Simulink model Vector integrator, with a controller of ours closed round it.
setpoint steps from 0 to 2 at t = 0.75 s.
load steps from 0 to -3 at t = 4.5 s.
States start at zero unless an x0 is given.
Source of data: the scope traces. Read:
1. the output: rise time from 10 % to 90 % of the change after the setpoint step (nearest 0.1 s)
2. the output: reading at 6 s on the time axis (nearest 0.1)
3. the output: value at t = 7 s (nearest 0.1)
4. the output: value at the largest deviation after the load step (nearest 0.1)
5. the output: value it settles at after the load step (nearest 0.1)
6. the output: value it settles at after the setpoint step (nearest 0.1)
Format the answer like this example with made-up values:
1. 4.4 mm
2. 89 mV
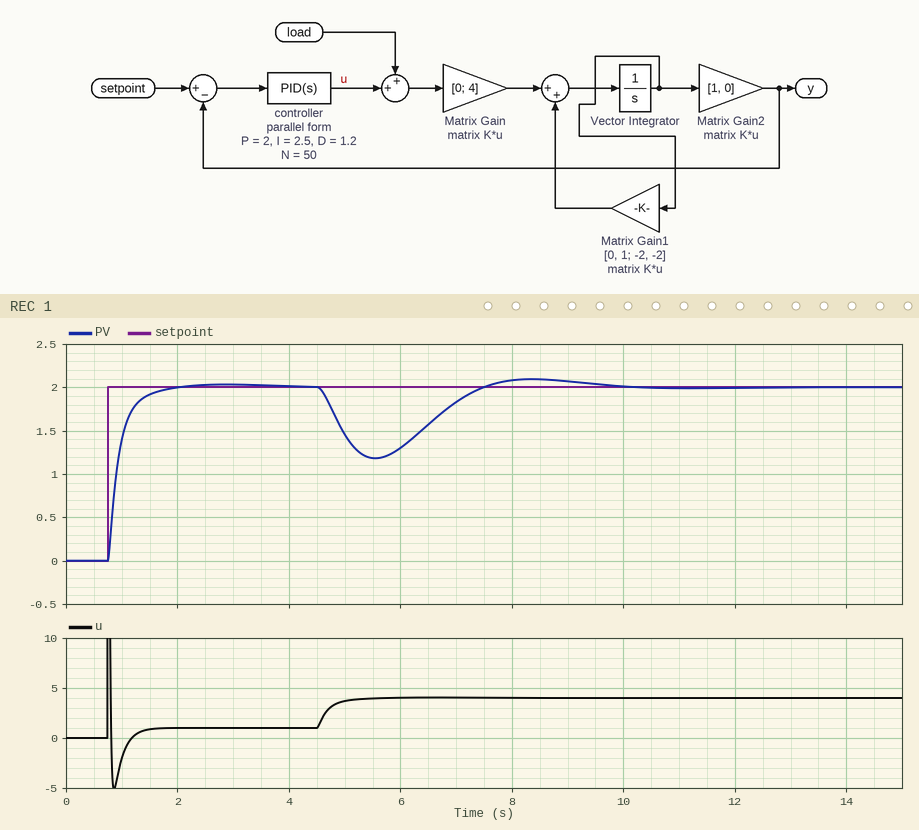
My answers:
1. 0.5 s
2. 1.3
3. 1.8
4. 1.2
5. 2.0
6. 2.0
